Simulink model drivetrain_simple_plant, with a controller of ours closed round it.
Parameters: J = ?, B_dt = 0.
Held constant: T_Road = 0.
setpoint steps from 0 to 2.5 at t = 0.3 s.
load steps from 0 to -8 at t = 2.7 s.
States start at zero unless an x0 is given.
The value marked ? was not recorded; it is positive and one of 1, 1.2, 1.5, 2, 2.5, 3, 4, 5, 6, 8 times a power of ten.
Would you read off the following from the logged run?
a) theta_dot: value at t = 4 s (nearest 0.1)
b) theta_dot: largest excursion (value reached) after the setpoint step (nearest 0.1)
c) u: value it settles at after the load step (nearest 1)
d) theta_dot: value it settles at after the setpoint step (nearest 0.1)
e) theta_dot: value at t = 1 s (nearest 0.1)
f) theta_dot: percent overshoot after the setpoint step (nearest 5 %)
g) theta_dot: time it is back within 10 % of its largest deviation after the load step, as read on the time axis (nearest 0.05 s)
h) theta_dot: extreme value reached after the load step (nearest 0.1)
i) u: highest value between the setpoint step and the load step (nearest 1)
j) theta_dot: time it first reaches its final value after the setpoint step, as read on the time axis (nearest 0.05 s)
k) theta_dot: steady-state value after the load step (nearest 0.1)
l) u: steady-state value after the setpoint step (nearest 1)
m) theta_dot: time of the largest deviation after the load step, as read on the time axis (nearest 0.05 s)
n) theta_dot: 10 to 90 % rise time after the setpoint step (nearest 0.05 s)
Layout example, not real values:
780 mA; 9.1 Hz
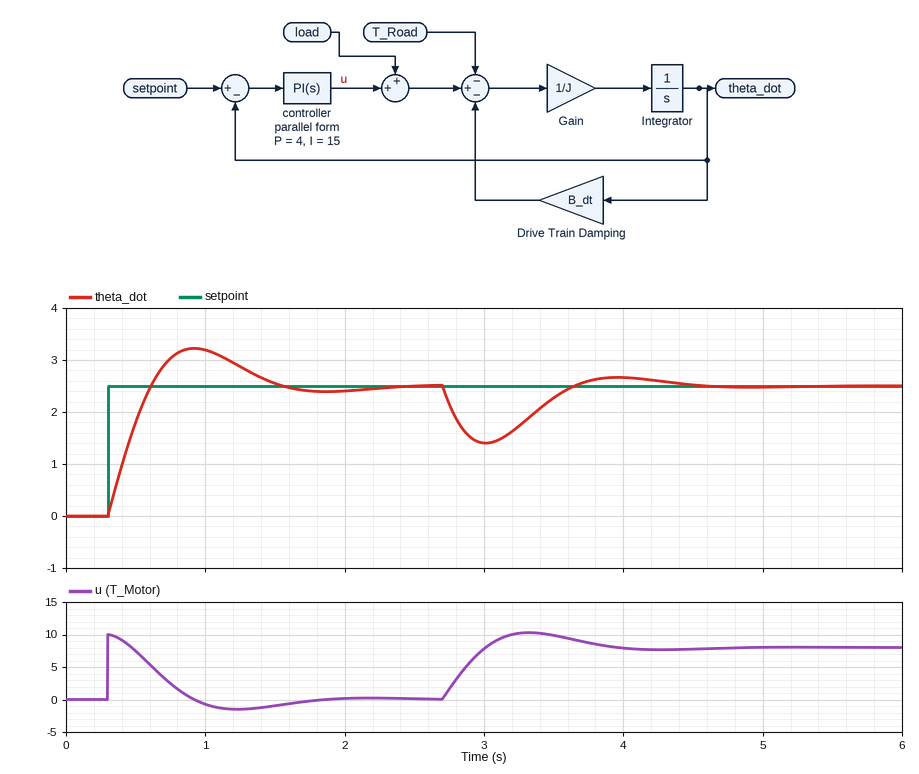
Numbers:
2.7; 3.2; 8; 2.5; 3.2; 30 %; 4.20 s; 1.4; 10; 0.60 s; 2.5; 0; 3.00 s; 0.25 s
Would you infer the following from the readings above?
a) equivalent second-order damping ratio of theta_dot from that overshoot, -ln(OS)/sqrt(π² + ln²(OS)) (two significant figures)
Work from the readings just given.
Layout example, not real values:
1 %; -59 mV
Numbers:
0.36
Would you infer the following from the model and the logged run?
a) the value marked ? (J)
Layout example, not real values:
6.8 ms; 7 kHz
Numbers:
1
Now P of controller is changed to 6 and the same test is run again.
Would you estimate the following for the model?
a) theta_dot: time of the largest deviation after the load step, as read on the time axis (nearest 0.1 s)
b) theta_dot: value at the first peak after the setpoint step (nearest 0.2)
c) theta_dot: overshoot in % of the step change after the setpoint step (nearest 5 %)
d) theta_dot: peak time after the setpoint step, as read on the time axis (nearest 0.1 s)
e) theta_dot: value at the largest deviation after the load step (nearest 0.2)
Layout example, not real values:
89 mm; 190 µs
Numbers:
3.0 s; 3.0; 20 %; 0.9 s; 1.6
